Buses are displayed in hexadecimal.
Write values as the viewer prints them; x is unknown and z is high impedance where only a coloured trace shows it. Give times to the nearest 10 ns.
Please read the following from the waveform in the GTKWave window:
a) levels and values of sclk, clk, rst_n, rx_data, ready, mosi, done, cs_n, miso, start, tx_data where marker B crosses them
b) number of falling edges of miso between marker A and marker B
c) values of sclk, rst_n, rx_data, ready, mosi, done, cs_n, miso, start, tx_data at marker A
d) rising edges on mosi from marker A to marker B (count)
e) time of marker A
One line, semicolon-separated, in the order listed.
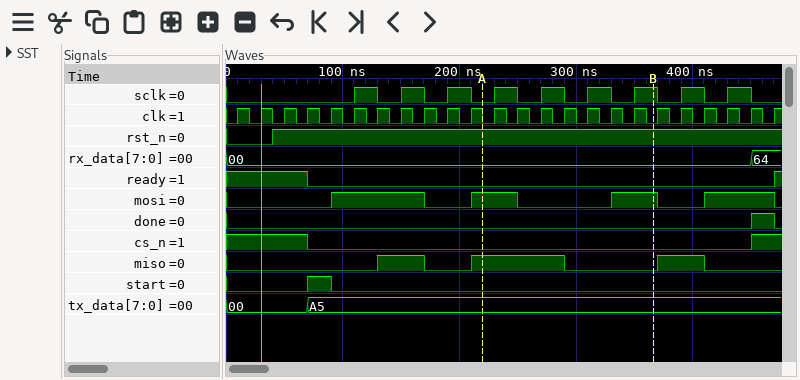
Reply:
sclk=1, clk=0, rst_n=1, rx_data=00, ready=0, mosi=1, done=0, cs_n=0, miso=0, start=0, tx_data=A5; 1; sclk=0, rst_n=1, rx_data=00, ready=0, mosi=1, done=0, cs_n=0, miso=1, start=0, tx_data=A5; 1; 220 ns
